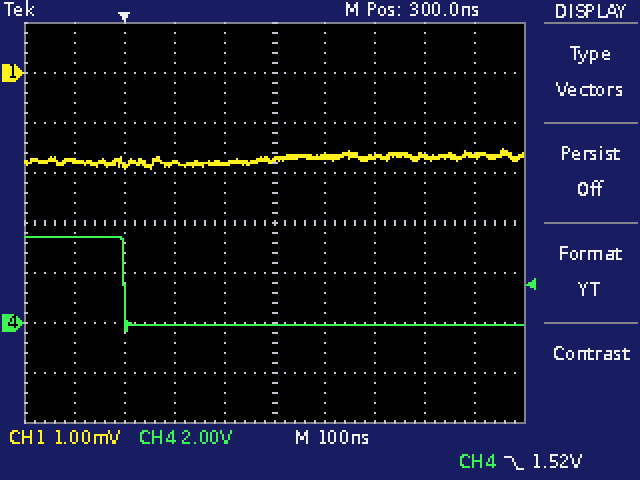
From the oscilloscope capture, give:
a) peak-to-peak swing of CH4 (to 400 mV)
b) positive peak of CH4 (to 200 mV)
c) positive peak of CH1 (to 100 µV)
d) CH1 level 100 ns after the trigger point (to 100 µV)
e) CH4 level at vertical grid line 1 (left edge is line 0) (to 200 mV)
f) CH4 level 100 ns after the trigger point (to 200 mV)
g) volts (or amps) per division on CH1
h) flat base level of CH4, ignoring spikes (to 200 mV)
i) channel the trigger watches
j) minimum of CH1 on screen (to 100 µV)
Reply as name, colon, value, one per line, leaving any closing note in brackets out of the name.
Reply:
peak-to-peak swing of CH4: 3.6 V
positive peak of CH4: 3.4 V
positive peak of CH1: -1.5 mV
CH1 level 100 ns after the trigger point: -1.8 mV
CH4 level at vertical grid line 1 (left edge is line 0): 3.4 V
CH4 level 100 ns after the trigger point: 0.0 V
volts (or amps) per division on CH1: 1 mV
flat base level of CH4, ignoring spikes: 0.0 V
channel the trigger watches: CH4
minimum of CH1 on screen: -1.9 mV
